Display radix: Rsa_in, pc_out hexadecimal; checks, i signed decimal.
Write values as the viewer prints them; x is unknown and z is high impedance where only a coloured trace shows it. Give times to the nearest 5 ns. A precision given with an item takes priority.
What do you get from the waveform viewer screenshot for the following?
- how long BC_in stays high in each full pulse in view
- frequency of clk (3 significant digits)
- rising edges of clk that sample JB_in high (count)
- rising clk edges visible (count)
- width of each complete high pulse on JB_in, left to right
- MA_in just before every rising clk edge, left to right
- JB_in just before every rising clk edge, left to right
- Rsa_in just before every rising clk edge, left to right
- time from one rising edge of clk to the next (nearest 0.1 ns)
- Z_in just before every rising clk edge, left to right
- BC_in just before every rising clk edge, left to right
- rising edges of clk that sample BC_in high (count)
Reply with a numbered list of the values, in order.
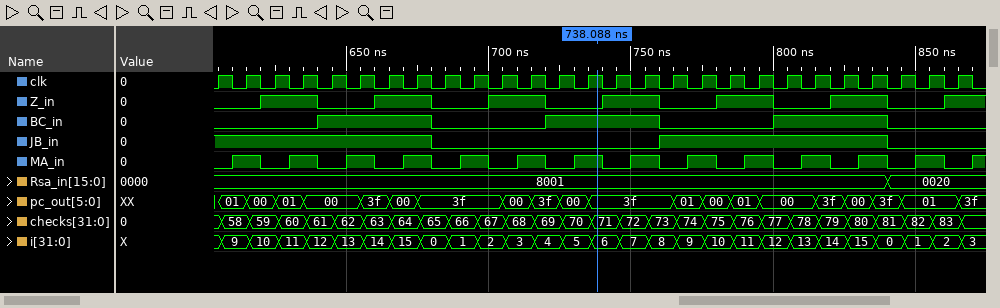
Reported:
1. 40 ns, 40 ns, 40 ns
2. 100 MHz
3. 16
4. 27
5. 80 ns
6. 0 1 0 1 0 1 0 1 0 1 0 1 0 1 0 1 0 1 0 1 0 1 0 1 0 1 0
7. 1 1 1 1 1 1 1 1 0 0 0 0 0 0 0 0 1 1 1 1 1 1 1 1 0 0 0
8. 8001, 8001, 8001, 8001, 8001, 8001, 8001, 8001, 8001, 8001, 8001, 8001, 8001, 8001, 8001, 8001, 8001, 8001, 8001, 8001, 8001, 8001, 8001, 8001, 0020, 0020, 0020
9. 10 ns
10. 0 0 1 1 0 0 1 1 0 0 1 1 0 0 1 1 0 0 1 1 0 0 1 1 0 0 1
11. 0 0 0 0 1 1 1 1 0 0 0 0 1 1 1 1 0 0 0 0 1 1 1 1 0 0 0
12. 12
